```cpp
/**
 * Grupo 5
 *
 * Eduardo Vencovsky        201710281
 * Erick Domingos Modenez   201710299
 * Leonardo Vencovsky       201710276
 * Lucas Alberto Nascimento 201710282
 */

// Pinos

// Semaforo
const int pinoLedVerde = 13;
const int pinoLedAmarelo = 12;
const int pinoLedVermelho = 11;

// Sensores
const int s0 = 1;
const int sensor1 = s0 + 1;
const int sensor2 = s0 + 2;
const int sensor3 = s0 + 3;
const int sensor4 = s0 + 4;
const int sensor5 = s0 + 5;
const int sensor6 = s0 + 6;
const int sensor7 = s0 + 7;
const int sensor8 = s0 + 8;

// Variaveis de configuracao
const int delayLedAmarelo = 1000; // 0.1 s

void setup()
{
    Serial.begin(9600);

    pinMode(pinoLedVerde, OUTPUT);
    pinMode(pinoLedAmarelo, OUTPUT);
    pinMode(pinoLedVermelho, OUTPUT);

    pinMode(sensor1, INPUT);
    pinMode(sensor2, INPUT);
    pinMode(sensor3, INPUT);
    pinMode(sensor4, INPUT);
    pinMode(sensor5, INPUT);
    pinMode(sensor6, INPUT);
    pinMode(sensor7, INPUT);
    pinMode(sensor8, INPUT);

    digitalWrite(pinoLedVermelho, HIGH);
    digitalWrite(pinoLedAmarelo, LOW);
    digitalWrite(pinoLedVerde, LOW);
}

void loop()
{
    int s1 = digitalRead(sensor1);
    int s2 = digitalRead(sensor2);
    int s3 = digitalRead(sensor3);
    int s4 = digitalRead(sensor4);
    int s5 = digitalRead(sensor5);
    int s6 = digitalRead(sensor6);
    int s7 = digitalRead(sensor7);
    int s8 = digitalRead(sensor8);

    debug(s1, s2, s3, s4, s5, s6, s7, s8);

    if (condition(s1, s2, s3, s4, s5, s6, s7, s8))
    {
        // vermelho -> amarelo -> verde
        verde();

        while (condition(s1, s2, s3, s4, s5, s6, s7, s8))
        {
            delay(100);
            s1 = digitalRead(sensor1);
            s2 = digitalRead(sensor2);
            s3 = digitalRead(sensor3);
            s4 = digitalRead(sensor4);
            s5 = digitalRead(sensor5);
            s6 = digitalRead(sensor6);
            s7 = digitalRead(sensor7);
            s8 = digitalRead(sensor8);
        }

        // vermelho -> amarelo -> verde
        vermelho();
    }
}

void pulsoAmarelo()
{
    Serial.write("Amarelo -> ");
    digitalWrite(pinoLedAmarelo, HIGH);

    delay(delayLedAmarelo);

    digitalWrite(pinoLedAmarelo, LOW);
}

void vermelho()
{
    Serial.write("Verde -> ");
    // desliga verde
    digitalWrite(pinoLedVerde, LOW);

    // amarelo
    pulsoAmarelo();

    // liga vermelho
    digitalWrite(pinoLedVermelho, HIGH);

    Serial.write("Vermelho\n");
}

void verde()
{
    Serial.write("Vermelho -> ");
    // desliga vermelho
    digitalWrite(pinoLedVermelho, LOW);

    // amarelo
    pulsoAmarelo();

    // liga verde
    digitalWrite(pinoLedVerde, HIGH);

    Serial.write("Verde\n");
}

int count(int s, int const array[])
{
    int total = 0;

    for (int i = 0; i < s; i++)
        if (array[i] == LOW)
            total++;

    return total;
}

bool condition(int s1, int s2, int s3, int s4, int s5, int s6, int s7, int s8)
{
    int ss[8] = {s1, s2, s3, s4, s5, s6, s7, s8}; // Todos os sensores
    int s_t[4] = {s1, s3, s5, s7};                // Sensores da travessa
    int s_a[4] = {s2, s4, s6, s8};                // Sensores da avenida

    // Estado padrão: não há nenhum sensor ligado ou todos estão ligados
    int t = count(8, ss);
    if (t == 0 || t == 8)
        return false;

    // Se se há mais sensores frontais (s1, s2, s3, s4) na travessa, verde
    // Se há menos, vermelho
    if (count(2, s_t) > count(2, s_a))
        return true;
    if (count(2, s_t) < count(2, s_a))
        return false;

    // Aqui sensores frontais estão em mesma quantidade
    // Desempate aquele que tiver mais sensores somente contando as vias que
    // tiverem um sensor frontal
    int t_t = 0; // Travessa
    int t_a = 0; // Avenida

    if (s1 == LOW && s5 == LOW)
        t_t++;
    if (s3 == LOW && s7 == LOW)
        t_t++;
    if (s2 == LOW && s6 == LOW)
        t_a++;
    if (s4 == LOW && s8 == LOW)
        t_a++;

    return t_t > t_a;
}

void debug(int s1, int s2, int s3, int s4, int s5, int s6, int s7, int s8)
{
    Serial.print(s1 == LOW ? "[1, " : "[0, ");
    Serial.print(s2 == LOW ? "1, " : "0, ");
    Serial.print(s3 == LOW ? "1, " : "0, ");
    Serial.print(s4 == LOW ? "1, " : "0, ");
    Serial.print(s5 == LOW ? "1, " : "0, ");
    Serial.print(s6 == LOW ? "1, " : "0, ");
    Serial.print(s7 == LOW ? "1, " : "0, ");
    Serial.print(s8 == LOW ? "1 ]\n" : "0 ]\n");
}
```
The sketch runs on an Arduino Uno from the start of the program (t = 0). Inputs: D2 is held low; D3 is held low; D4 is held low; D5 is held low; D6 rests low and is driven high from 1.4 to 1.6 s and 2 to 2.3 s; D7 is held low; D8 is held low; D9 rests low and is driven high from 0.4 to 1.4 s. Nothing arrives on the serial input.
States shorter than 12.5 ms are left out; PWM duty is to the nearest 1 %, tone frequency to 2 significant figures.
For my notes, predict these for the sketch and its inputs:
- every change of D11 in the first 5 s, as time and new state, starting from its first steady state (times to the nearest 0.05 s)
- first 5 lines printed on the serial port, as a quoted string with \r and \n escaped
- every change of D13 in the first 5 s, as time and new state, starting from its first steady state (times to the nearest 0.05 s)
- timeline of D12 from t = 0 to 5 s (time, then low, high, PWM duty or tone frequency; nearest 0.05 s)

0 s high; 0.45 s low; 2.55 s high
"[1, 1, 1, 1, 1, 1, 1, 1 ]\n[1, 1, 1, 1, 1, 1, 1, 1 ]\n[1, 1, 1, 1, 1, 1, 1, 1 ]\n[1, 1, 1, 1, 1, 1, 1, 1 ]\n[1, 1, 1, 1, 1, 1, 1, 1 ]\n"
0 s low; 1.45 s high; 1.55 s low
0 s low; 0.45 s high; 1.45 s low; 1.55 s high; 2.55 s low
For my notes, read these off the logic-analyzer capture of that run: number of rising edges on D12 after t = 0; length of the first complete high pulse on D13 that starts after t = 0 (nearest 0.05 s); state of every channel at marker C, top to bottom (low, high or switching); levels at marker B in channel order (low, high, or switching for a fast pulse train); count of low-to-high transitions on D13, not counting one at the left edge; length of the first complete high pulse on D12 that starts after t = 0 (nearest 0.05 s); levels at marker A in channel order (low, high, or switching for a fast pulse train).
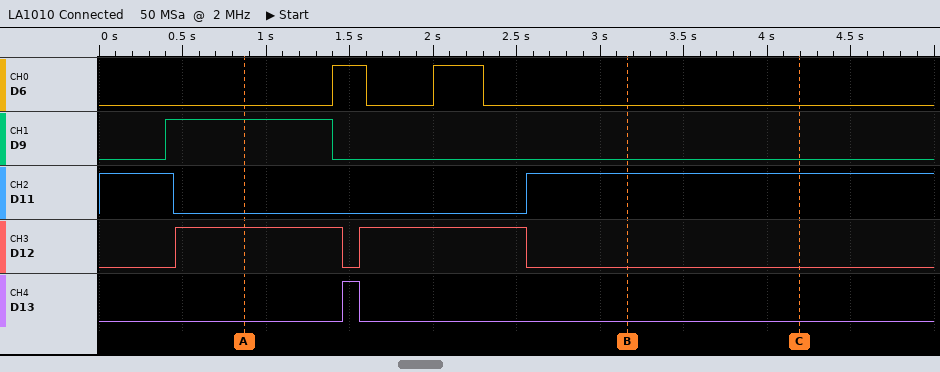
2
0.10 s
D6 low, D9 low, D11 high, D12 low, D13 low
D6 low, D9 low, D11 high, D12 low, D13 low
1
1.00 s
D6 low, D9 high, D11 low, D12 high, D13 low
